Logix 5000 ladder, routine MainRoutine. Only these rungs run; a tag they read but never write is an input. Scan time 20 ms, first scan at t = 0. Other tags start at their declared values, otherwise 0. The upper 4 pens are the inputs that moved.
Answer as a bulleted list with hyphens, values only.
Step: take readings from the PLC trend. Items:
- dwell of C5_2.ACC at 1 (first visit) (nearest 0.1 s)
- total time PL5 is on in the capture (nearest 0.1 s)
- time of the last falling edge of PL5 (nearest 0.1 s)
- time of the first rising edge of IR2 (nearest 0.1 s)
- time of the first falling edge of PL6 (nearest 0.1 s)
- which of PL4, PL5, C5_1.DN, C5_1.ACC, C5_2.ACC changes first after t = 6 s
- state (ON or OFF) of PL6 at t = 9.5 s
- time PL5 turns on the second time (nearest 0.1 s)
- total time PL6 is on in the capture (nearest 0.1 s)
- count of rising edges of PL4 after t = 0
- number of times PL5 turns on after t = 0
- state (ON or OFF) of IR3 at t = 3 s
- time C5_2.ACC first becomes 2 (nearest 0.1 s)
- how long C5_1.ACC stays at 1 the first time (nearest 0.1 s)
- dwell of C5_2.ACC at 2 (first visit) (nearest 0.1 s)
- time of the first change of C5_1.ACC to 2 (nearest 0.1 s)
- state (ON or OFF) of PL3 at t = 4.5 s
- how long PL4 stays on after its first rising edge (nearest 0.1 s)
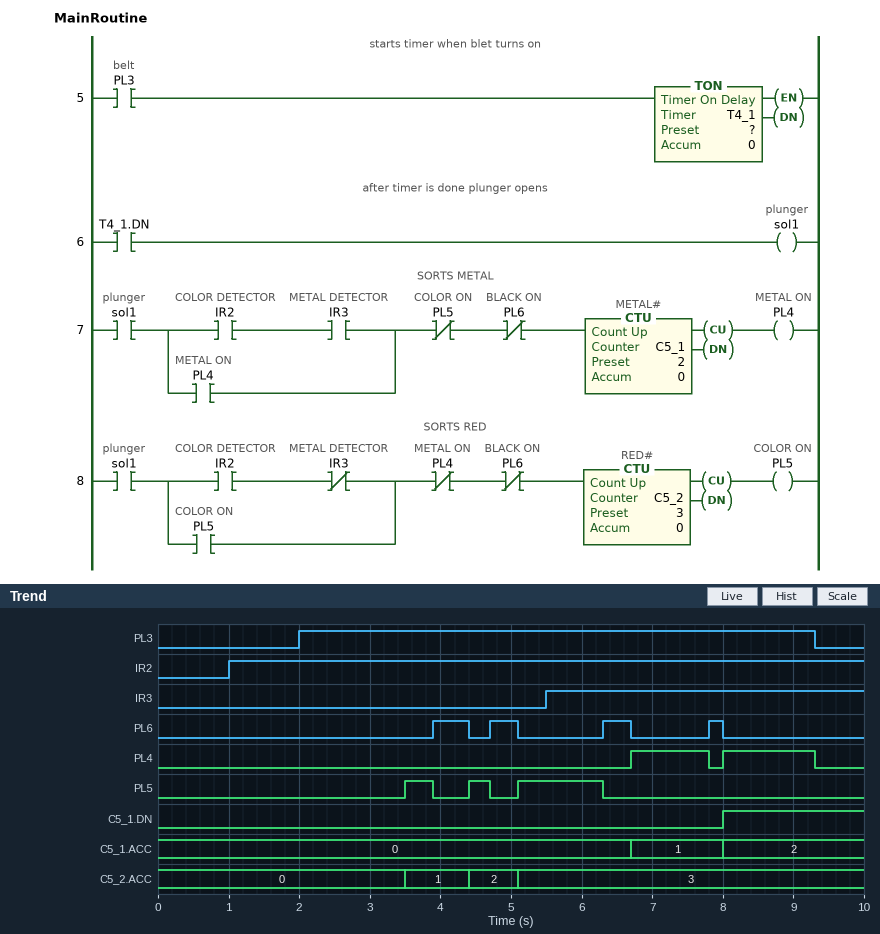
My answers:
- 0.9 s
- 1.9 s
- 6.3 s
- 1.0 s
- 4.4 s
- PL5
- OFF
- 4.4 s
- 1.5 s
- 2
- 3
- OFF
- 4.4 s
- 1.3 s
- 0.7 s
- 8.0 s
- ON
- 1.1 s
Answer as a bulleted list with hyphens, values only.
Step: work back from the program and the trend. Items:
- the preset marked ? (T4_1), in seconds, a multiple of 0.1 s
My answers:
- 1.5 s
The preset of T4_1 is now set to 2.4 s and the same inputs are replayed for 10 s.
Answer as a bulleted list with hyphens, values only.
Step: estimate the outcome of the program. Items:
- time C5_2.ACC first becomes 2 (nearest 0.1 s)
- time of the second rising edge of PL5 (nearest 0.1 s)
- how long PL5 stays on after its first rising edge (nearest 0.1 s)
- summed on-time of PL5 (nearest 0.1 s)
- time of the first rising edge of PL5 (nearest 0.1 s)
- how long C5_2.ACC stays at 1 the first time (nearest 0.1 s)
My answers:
- 5.1 s
- 5.1 s
- 0.3 s
- 1.5 s
- 4.4 s
- 0.7 s
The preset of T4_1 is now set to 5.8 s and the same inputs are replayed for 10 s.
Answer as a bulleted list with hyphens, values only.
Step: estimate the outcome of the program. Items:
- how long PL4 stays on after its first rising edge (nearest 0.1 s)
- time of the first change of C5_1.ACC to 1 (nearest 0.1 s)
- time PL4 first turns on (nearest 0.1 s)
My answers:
- 1.3 s
- 8.0 s
- 8.0 s
